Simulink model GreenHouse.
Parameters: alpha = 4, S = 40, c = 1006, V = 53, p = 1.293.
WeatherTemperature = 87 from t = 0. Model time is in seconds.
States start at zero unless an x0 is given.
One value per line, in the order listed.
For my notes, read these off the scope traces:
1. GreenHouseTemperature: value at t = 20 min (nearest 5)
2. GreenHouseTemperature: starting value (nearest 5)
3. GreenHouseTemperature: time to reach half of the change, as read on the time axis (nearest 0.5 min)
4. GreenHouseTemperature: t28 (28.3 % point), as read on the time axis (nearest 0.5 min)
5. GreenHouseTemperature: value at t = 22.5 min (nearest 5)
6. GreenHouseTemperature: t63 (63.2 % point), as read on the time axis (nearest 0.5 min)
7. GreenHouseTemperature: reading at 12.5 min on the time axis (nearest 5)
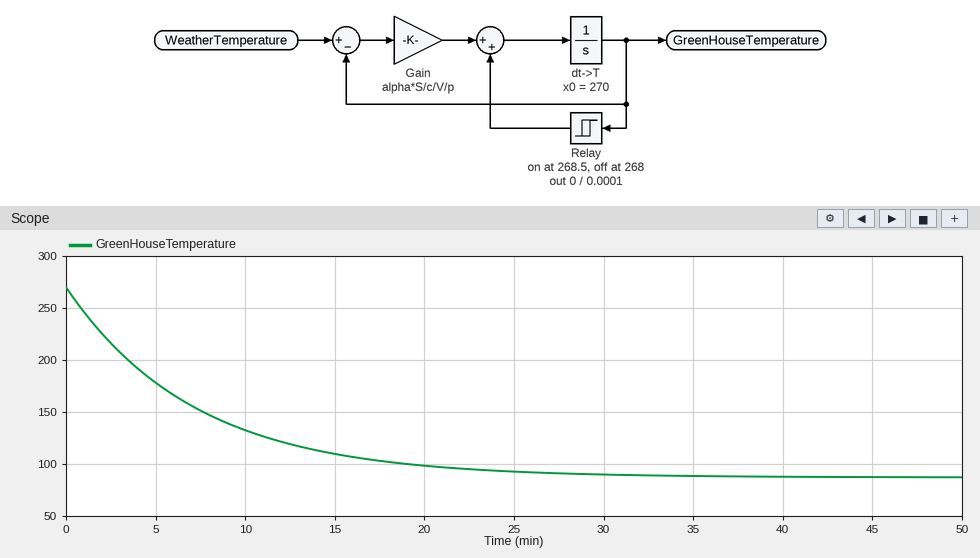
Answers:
100
270
5.0 min
2.5 min
95
7.0 min
120
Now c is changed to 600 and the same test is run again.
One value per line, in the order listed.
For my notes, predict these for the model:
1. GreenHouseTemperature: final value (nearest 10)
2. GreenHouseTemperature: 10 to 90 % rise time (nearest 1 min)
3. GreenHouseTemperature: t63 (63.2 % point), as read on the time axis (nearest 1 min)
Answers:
90
9 min
4 min
